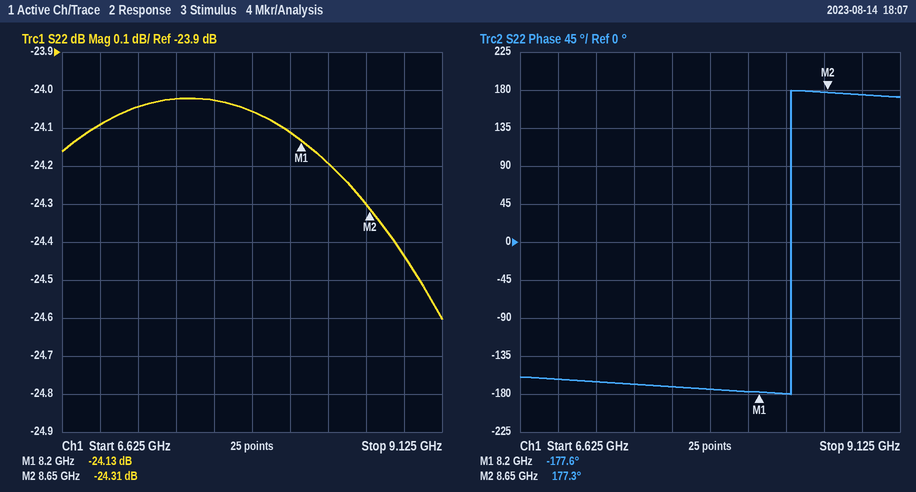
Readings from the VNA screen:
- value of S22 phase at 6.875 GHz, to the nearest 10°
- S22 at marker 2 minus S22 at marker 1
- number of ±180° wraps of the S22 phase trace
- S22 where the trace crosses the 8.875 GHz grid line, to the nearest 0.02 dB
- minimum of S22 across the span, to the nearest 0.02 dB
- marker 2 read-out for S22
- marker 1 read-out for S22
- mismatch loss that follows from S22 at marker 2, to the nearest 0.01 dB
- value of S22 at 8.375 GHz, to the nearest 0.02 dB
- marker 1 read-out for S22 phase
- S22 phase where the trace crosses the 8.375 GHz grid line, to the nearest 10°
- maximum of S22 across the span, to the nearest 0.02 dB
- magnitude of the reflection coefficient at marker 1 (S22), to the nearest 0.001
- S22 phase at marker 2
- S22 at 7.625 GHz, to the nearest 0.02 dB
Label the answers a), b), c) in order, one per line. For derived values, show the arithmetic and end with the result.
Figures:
a) -160°
b) -24.31 − (-24.13) = -0.18 dB
c) 1
d) -24.44 dB
e) -24.60 dB
f) -24.31 dB
g) -24.13 dB
h) −10 log10(1 − 10^(-24.31/10)) ≈ 0.02 dB
i) -24.20 dB
j) -177.6°
k) -180°
l) -24.02 dB
m) 10^(-24.13/20) ≈ 0.062
n) 177.3°
o) -24.02 dB
